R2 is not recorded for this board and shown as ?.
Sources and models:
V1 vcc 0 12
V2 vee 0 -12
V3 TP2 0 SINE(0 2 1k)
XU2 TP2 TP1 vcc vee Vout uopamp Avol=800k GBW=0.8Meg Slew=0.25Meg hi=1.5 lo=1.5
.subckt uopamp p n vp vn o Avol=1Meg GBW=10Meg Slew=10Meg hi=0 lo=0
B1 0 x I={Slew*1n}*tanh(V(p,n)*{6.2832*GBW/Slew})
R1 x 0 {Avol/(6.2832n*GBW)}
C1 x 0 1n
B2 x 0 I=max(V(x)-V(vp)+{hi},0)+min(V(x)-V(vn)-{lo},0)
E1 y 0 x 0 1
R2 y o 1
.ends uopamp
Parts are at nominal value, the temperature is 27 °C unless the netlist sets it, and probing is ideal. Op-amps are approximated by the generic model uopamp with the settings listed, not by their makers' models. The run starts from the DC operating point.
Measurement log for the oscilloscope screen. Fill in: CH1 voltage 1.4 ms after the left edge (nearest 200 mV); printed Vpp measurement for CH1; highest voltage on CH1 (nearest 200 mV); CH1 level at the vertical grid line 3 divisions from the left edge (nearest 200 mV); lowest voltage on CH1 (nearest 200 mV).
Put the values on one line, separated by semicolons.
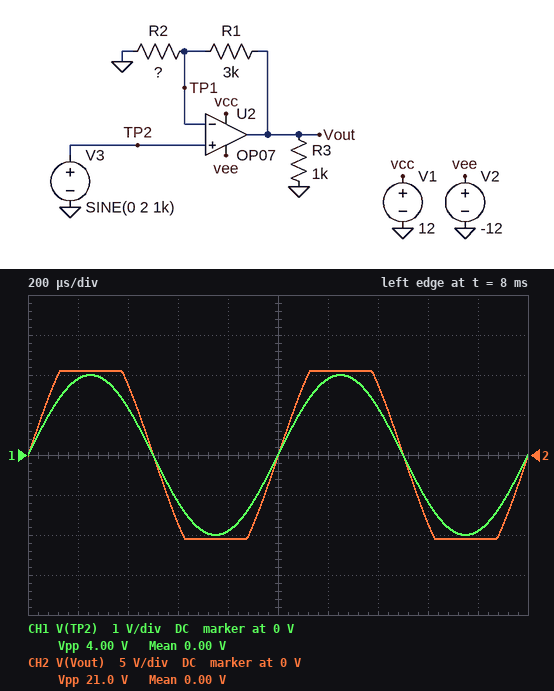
1.2 V; 4.00 V; 2.0 V; -1.2 V; -2.0 V
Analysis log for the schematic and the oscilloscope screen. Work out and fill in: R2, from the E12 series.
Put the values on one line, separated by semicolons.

470 Ω
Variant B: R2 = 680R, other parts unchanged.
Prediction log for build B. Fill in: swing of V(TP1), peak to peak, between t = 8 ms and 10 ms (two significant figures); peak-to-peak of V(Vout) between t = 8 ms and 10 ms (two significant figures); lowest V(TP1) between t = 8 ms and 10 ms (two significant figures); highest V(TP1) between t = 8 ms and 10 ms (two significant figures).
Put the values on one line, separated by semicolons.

3.9 V; 21 V; -1.9 V; 1.9 V
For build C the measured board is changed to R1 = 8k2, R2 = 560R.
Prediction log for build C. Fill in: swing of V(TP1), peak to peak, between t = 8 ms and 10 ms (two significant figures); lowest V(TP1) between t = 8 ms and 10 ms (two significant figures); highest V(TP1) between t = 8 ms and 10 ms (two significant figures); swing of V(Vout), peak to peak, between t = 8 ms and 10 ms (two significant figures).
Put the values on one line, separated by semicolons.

1.3 V; -670 mV; 670 mV; 21 V
